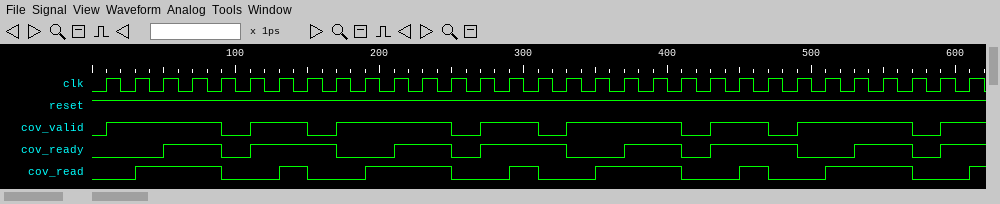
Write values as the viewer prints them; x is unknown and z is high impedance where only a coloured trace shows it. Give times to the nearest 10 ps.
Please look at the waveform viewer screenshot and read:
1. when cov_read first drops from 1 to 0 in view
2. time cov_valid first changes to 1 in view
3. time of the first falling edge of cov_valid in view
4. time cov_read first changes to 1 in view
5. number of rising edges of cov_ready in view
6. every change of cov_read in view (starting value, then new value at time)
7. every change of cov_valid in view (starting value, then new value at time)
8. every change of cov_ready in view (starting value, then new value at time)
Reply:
90 ps
10 ps
90 ps
30 ps
8
0, 1 at 30 ps, 0 at 90 ps, 1 at 130 ps, 0 at 150 ps, 1 at 190 ps, 0 at 250 ps, 1 at 290 ps, 0 at 310 ps, 1 at 350 ps, 0 at 410 ps, 1 at 450 ps, 0 at 470 ps, 1 at 510 ps, 0 at 570 ps, 1 at 610 ps
0, 1 at 10 ps, 0 at 90 ps, 1 at 110 ps, 0 at 150 ps, 1 at 170 ps, 0 at 250 ps, 1 at 270 ps, 0 at 310 ps, 1 at 330 ps, 0 at 410 ps, 1 at 430 ps, 0 at 470 ps, 1 at 490 ps, 0 at 570 ps, 1 at 590 ps
0, 1 at 50 ps, 0 at 90 ps, 1 at 110 ps, 0 at 170 ps, 1 at 210 ps, 0 at 250 ps, 1 at 270 ps, 0 at 330 ps, 1 at 370 ps, 0 at 410 ps, 1 at 430 ps, 0 at 490 ps, 1 at 530 ps, 0 at 570 ps, 1 at 590 ps
